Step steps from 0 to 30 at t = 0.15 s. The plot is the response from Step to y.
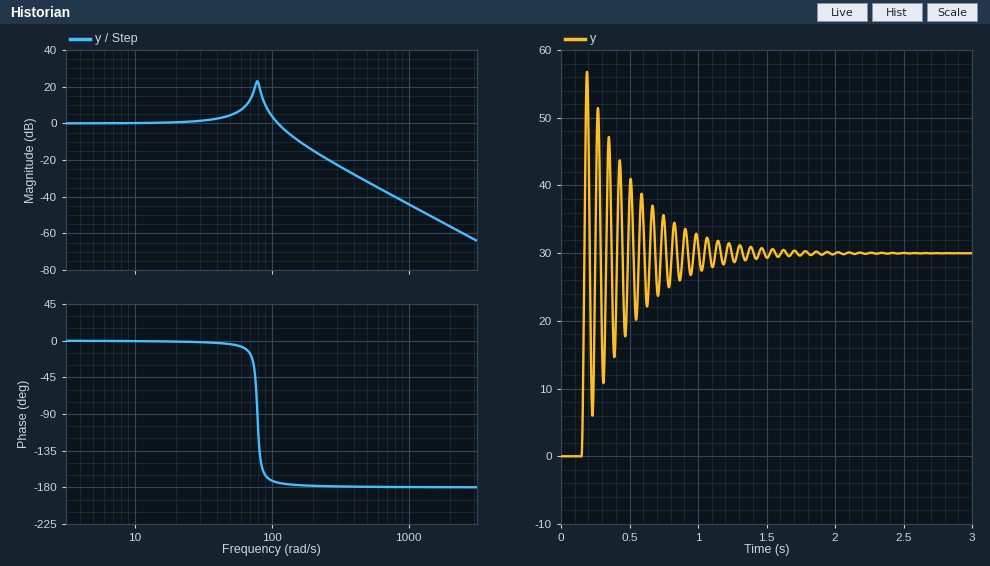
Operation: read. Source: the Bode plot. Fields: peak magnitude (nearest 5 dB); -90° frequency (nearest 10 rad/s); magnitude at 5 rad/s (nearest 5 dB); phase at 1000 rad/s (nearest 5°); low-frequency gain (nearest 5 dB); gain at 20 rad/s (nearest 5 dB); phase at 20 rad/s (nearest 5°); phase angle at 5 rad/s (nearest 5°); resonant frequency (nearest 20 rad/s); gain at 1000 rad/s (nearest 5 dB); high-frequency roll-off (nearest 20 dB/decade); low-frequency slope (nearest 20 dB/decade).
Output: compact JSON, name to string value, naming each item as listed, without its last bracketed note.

{"peak magnitude": "25 dB", "-90° frequency": "80 rad/s", "magnitude at 5 rad/s": "0 dB", "phase at 1000 rad/s": "-180°", "low-frequency gain": "0 dB", "gain at 20 rad/s": "0 dB", "phase at 20 rad/s": "0°", "phase angle at 5 rad/s": "0°", "resonant frequency": "80 rad/s", "gain at 1000 rad/s": "-45 dB", "high-frequency roll-off": "-40 dB/decade", "low-frequency slope": "0 dB/decade"}
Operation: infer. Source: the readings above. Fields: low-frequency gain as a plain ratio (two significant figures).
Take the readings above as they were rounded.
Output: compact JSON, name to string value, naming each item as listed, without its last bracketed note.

{"low-frequency gain as a plain ratio": "1.0"}
